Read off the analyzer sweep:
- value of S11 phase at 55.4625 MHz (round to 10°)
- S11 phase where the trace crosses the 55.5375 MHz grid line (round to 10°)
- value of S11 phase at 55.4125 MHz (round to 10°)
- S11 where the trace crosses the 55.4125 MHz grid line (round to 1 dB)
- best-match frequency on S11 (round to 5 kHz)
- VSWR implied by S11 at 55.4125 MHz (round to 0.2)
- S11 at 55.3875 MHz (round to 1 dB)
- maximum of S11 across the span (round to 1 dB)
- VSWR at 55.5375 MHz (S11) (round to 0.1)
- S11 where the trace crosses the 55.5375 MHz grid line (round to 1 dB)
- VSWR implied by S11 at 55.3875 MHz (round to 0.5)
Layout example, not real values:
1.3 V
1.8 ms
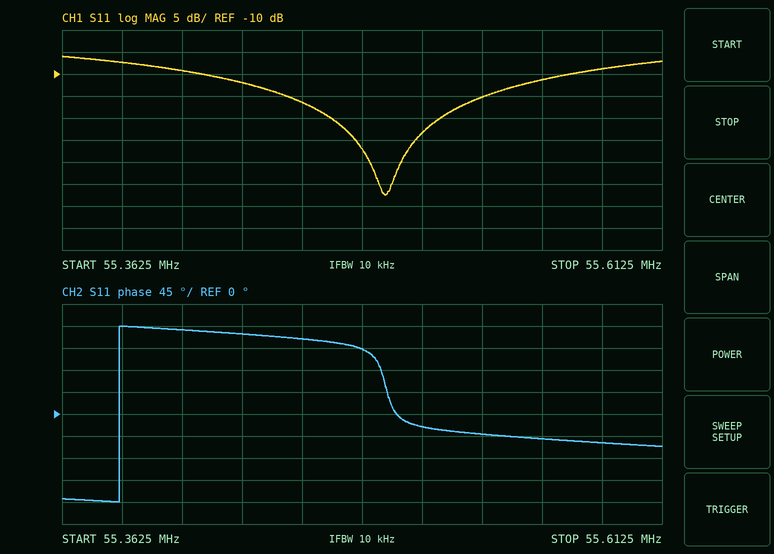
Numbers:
150°
-40°
170°
-9 dB
55.495 MHz
2.0
-7 dB
-6 dB
1.4
-15 dB
2.5
